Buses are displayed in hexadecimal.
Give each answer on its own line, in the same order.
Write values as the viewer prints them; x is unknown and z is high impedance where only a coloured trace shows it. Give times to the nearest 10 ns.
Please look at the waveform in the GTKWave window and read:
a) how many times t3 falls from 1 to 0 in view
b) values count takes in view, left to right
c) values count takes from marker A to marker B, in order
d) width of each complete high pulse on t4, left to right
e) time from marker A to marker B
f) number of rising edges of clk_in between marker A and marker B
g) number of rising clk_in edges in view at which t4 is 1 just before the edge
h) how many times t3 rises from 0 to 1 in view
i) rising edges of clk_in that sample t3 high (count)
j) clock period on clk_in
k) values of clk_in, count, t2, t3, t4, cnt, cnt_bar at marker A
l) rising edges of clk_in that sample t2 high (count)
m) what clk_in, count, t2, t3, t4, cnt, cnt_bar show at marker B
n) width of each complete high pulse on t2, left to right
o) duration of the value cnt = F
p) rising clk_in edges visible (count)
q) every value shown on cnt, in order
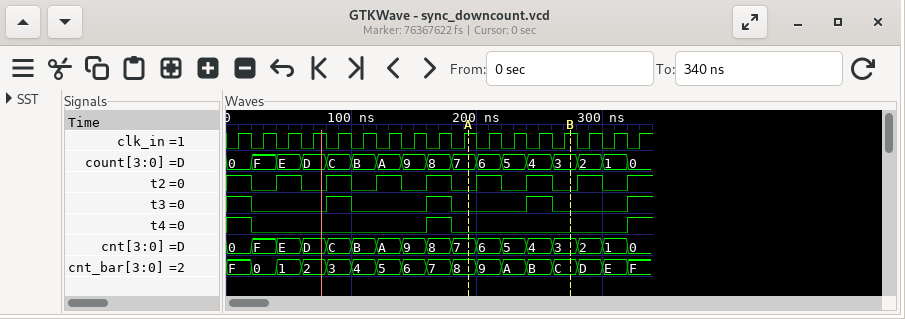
4
0, F, E, D, C, B, A, 9, 8, 7, 6, 5, 4, 3, 2, 1, 0
7, 6, 5, 4, 3
20 ns
80 ns
4
3
4
5
20 ns
clk_in=1, count=7, t2=0, t3=0, t4=0, cnt=7, cnt_bar=8
9
clk_in=1, count=3, t2=0, t3=0, t4=0, cnt=3, cnt_bar=C
20 ns, 20 ns, 20 ns, 20 ns, 20 ns, 20 ns, 20 ns
20 ns
17
0, F, E, D, C, B, A, 9, 8, 7, 6, 5, 4, 3, 2, 1, 0
